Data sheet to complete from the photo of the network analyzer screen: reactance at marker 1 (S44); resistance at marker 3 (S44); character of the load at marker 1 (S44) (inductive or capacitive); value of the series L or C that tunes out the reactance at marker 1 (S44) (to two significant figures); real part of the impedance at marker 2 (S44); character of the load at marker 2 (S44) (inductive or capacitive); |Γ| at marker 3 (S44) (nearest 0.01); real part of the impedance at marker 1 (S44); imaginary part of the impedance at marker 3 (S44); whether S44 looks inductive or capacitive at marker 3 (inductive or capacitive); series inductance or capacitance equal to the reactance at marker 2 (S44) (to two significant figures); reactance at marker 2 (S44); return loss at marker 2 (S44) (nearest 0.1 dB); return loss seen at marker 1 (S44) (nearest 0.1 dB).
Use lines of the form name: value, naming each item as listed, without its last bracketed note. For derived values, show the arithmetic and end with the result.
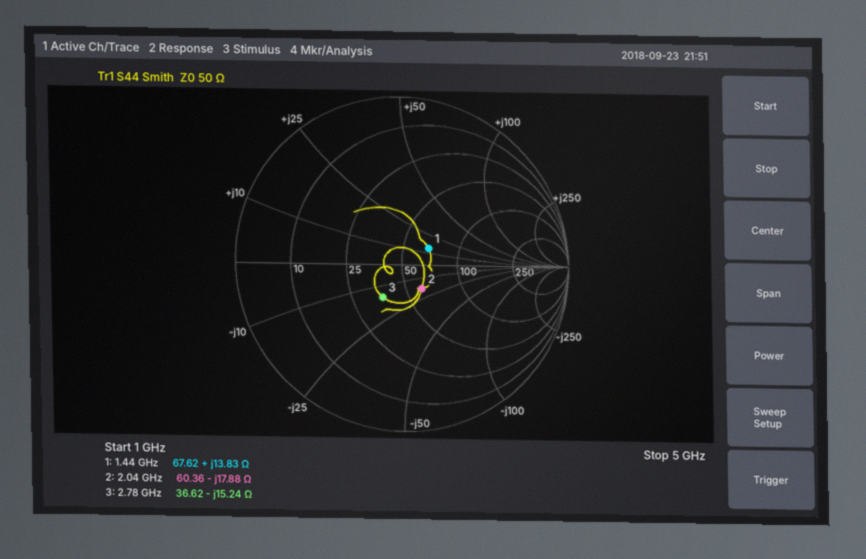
reactance at marker 1: +13.83 Ω
resistance at marker 3: 36.62 Ω
character of the load at marker 1 (S44): inductive
value of the series L or C that tunes out the reactance at marker 1 (S44): C = 1/(2π × 1.44 GHz × 13.83 Ω) ≈ 8.0 pF
real part of the impedance at marker 2: 60.36 Ω
character of the load at marker 2 (S44): capacitive
|Γ| at marker 3 (S44): 0.23
real part of the impedance at marker 1: 67.62 Ω
imaginary part of the impedance at marker 3: -15.24 Ω
whether S44 looks inductive or capacitive at marker 3: capacitive
series inductance or capacitance equal to the reactance at marker 2 (S44): C = 1/(2π × 2.04 GHz × 17.88 Ω) ≈ 4.4 pF
reactance at marker 2: -17.88 Ω
return loss at marker 2 (S44): 14.7 dB
return loss seen at marker 1 (S44): 14.5 dB
